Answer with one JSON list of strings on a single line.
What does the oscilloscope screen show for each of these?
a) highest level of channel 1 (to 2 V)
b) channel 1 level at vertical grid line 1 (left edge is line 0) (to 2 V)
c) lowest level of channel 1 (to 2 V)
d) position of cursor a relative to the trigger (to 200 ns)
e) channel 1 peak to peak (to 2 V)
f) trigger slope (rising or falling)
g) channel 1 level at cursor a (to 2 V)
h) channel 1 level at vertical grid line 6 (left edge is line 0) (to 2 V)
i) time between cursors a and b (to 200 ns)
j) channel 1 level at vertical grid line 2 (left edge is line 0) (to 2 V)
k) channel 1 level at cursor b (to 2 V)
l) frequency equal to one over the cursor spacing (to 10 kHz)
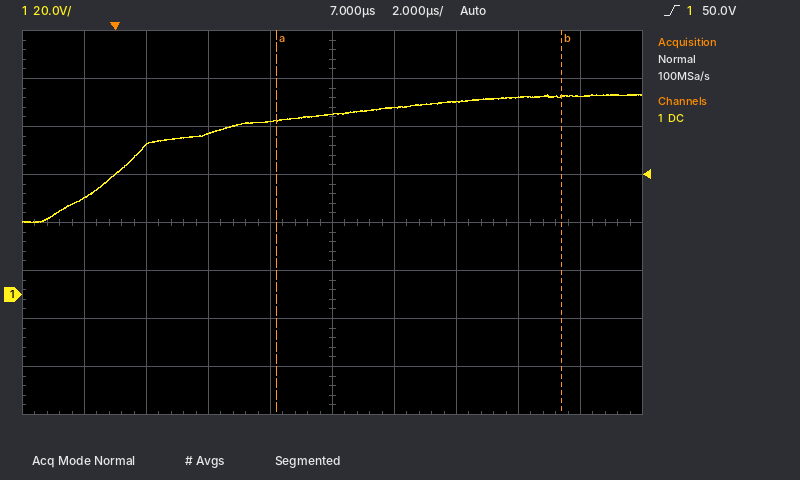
["84 V", "40 V", "30 V", "+5.2 µs", "54 V", "rising", "72 V", "78 V", "9.2 µs", "62 V", "82 V", "110 kHz"]
